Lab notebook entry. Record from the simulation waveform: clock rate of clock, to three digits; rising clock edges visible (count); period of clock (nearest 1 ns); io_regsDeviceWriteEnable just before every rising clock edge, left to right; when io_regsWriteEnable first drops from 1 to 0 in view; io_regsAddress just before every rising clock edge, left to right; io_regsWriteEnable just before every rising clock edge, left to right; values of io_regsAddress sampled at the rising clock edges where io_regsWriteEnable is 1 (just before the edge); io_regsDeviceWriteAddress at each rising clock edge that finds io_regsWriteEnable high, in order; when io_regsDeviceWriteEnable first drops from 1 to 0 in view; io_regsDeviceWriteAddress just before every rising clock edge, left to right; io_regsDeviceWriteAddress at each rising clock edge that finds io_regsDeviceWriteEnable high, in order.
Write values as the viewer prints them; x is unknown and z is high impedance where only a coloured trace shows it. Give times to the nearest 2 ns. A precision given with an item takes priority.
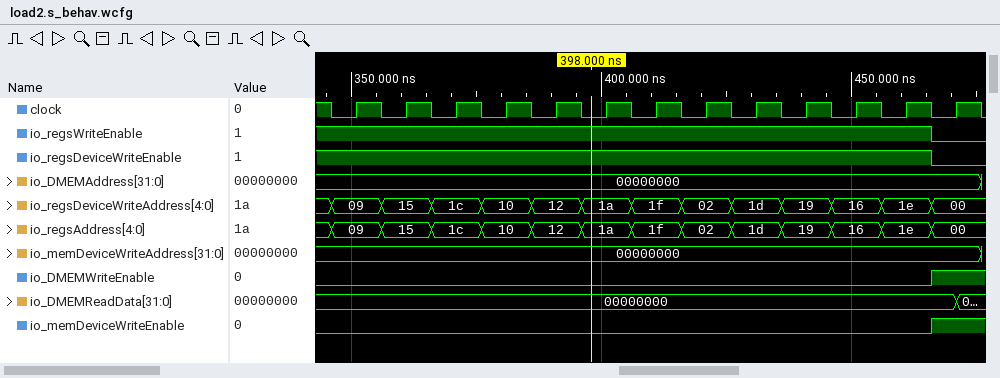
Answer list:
100 MHz
13
10 ns
1 1 1 1 1 1 1 1 1 1 1 1 0
466 ns
09, 15, 1c, 10, 12, 1a, 1f, 02, 1d, 19, 16, 1e, 00
1 1 1 1 1 1 1 1 1 1 1 1 0
09, 15, 1c, 10, 12, 1a, 1f, 02, 1d, 19, 16, 1e
09, 15, 1c, 10, 12, 1a, 1f, 02, 1d, 19, 16, 1e
466 ns
09, 15, 1c, 10, 12, 1a, 1f, 02, 1d, 19, 16, 1e, 00
09, 15, 1c, 10, 12, 1a, 1f, 02, 1d, 19, 16, 1e
